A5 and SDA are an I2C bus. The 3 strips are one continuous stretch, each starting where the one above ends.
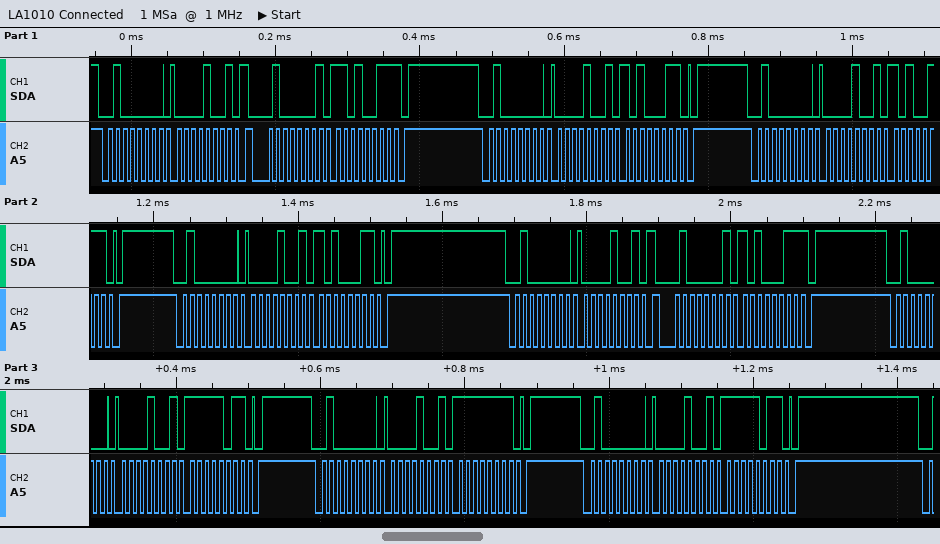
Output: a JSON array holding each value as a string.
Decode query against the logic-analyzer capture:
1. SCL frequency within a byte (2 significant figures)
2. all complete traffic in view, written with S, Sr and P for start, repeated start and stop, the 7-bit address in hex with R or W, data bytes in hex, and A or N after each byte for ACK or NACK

["100 kHz", "S 20W A 09 A Sr 20R A D3 N P S 20W A 09 A A3 A P S 20W A 09 A A7 A P S 20W A 09 A A3 A P S 20W A 09 A Sr 20R A A3 N P S 20W A 09 A FB A P S 20W A 09 A FF A P S 20W A 09 A FB A P"]
